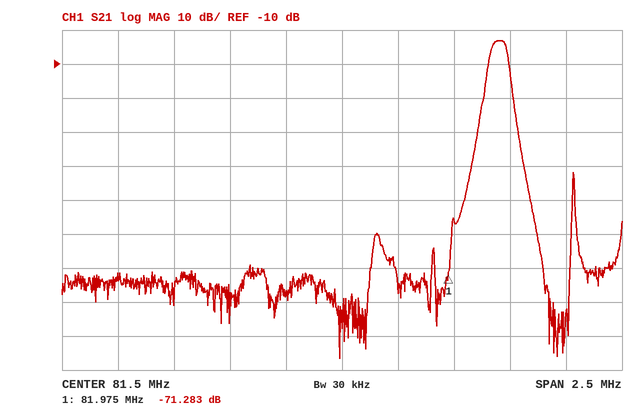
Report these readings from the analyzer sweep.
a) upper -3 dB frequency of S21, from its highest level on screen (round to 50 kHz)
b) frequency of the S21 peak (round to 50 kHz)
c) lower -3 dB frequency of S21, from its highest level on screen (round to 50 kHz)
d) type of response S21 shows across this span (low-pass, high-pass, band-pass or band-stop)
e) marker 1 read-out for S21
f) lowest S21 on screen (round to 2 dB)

82.25 MHz
82.20 MHz
82.15 MHz
band-pass
-71.283 dB
-96 dB
